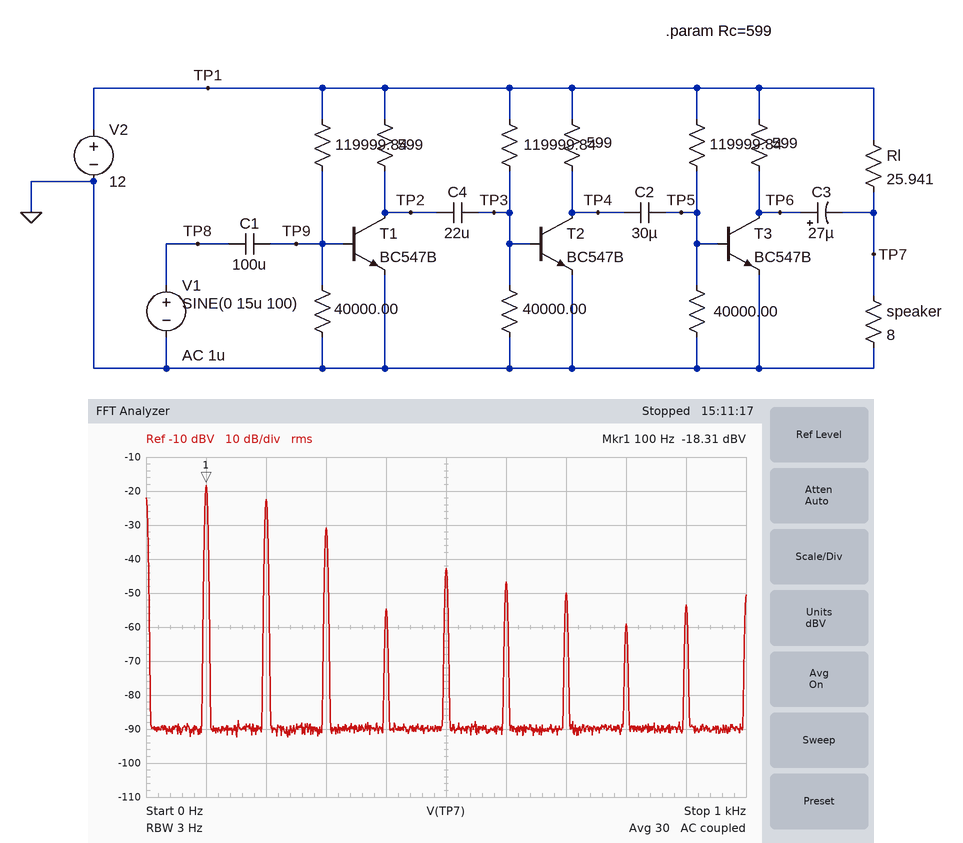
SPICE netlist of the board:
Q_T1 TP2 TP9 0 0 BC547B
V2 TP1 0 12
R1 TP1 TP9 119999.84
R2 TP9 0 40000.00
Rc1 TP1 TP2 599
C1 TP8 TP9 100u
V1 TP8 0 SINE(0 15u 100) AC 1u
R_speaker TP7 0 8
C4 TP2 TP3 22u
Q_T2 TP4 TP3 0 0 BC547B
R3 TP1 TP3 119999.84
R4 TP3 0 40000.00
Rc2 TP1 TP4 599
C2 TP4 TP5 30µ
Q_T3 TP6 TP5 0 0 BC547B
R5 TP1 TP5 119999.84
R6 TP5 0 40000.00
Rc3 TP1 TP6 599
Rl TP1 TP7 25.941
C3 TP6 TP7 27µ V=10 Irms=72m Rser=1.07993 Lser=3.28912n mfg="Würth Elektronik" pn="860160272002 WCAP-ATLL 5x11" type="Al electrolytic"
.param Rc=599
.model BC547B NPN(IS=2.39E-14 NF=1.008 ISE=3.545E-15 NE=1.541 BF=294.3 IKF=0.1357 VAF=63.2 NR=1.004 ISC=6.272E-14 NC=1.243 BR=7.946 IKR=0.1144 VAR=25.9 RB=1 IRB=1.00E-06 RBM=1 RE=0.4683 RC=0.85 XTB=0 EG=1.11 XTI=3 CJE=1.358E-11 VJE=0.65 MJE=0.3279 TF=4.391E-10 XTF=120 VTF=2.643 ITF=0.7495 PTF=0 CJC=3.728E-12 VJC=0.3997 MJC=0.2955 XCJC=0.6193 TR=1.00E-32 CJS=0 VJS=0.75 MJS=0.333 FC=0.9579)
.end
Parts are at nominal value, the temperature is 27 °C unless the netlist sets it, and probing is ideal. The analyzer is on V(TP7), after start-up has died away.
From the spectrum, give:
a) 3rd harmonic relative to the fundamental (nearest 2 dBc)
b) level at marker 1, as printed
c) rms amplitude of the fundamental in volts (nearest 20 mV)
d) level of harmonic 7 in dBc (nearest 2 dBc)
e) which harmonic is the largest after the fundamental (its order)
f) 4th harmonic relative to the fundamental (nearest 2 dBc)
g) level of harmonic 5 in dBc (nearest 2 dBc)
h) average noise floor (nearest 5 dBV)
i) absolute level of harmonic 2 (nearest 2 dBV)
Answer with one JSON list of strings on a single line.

["-12 dBc", "-18.31 dBV", "120 mV", "-32 dBc", "2", "-36 dBc", "-24 dBc", "-90 dBV", "-22 dBV"]
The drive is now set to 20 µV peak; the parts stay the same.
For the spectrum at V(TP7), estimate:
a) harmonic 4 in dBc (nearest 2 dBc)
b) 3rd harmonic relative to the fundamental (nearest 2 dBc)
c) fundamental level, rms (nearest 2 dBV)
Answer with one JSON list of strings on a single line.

["-22 dBc", "-10 dBc", "-18 dBV"]
